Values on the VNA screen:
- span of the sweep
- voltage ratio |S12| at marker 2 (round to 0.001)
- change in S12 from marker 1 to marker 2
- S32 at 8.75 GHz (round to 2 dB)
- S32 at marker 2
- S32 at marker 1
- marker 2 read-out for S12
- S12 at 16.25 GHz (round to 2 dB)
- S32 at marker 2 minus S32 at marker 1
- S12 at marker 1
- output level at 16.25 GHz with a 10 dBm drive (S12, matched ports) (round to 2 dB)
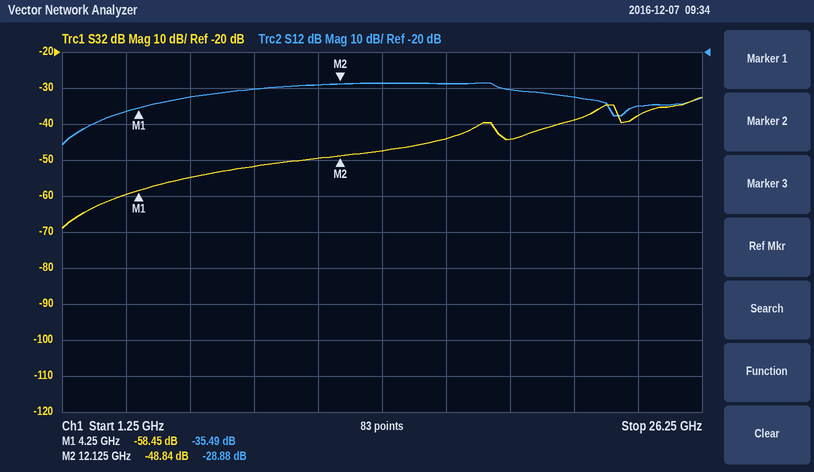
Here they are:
25 GHz
0.036
6.61 dB
-52 dB
-48.84 dB
-58.45 dB
-28.88 dB
-28 dB
9.61 dB
-35.49 dB
-18 dBm
